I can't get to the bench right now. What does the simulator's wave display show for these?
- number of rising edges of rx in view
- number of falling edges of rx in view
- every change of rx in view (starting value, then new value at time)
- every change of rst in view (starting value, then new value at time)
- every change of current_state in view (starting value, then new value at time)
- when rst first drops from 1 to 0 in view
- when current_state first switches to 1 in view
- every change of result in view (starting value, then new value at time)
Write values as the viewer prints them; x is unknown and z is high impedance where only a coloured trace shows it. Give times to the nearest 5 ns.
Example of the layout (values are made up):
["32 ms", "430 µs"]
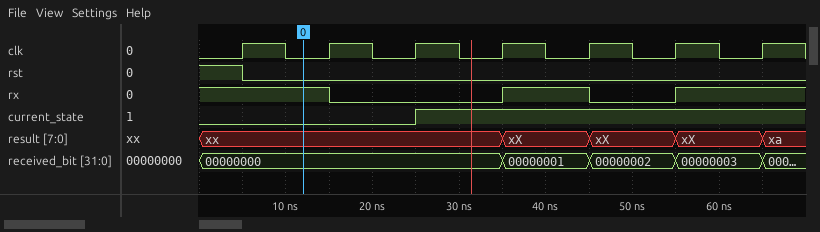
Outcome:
["2", "2", "1, 0 at 15 ns, 1 at 35 ns, 0 at 45 ns, 1 at 55 ns", "1, 0 at 5 ns", "0, 1 at 25 ns", "5 ns", "25 ns", "xx, xX at 35 ns, xX at 45 ns, xX at 55 ns, xa at 65 ns"]
